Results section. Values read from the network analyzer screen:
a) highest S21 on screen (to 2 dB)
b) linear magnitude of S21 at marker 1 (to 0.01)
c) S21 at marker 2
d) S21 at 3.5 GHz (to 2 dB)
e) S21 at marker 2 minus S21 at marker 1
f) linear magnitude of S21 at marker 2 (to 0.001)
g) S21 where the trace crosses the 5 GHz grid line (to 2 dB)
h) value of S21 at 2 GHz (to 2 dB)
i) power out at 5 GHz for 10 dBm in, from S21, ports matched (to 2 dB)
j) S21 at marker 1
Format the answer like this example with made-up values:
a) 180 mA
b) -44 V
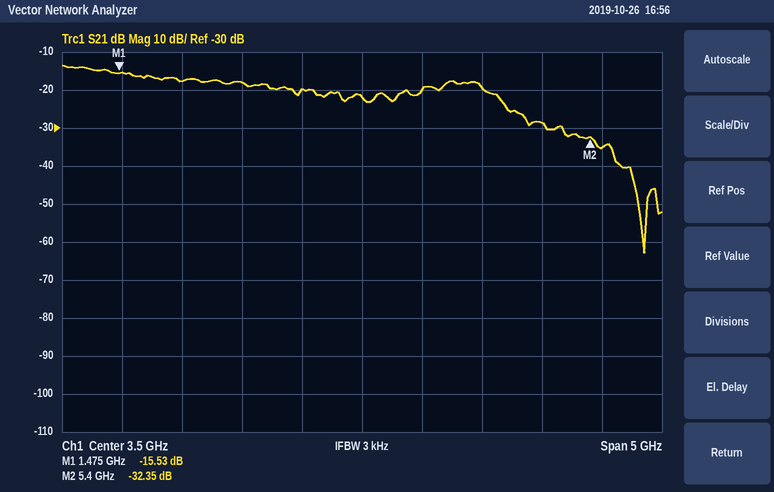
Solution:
a) -14 dB
b) 0.17
c) -32.35 dB
d) -22 dB
e) -16.82 dB
f) 0.024
g) -28 dB
h) -18 dB
i) -18 dBm
j) -15.53 dB
